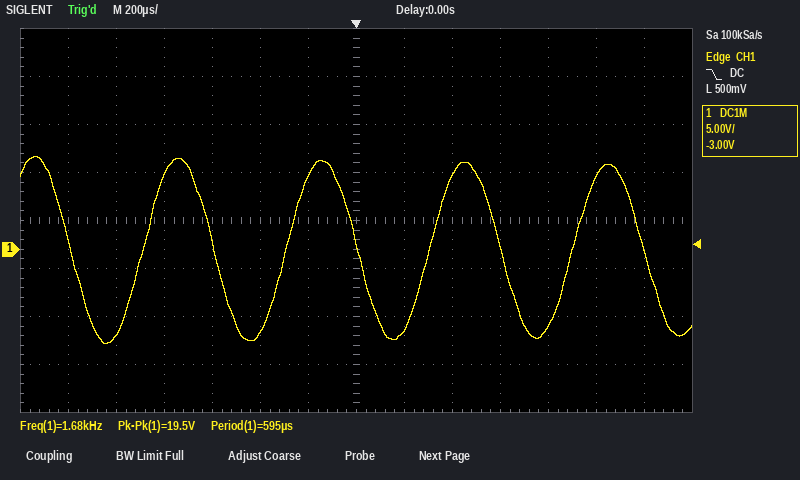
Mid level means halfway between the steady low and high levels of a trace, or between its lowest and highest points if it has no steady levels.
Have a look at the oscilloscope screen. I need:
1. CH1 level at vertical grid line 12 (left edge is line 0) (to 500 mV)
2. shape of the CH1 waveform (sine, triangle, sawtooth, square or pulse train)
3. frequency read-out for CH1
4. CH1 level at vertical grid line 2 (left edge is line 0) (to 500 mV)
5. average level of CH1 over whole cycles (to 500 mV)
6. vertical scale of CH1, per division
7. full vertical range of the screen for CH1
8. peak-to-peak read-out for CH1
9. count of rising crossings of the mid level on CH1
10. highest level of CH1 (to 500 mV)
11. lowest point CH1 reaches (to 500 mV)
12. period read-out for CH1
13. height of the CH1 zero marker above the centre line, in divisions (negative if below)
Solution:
7.5 V
sine
1.68 kHz
-9.0 V
0.0 V
5 V
40 V
19.5 V
4
9.5 V
-10.0 V
595 µs
-0.6 div
